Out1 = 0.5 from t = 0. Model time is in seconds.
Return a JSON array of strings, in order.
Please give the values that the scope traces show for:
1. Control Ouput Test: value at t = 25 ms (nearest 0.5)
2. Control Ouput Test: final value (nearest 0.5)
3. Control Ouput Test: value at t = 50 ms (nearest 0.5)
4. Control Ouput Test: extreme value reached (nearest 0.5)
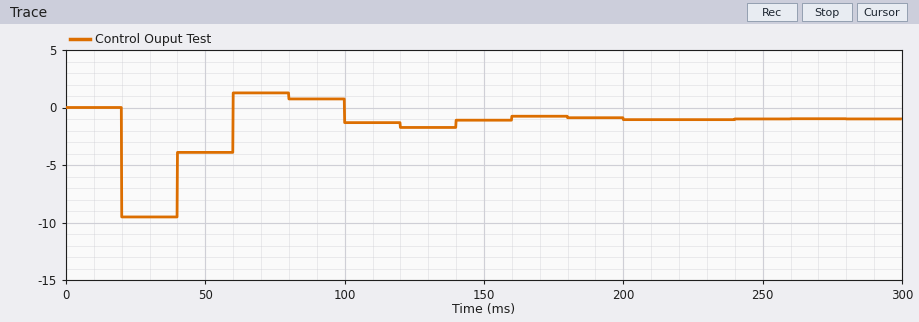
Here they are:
["-9.5", "-1.0", "-4.0", "-9.5"]
